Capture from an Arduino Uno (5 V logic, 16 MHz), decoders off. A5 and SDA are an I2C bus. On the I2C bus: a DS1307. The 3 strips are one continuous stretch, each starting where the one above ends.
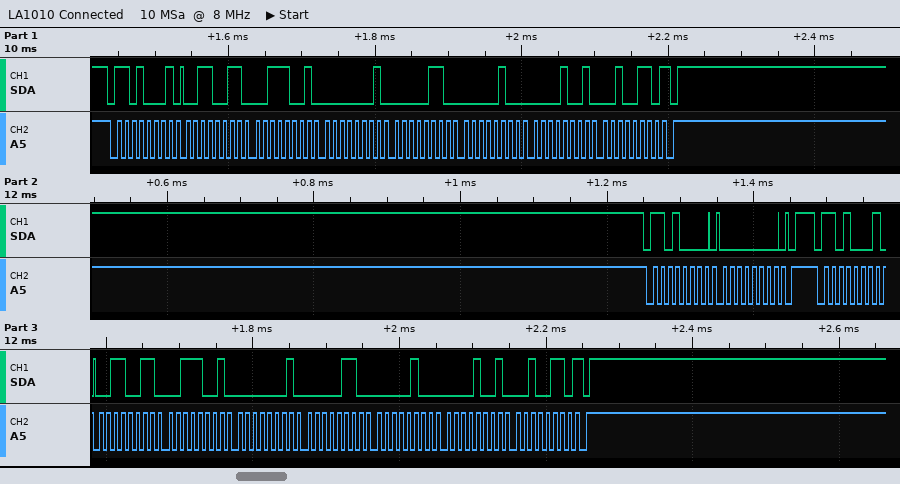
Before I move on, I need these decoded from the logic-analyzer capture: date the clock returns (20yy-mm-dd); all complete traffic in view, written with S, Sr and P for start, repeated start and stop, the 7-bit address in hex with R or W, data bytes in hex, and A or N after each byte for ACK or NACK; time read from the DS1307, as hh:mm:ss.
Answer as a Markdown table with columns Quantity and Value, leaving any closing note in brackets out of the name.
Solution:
| Quantity | Value |
|---|---|
| date the clock returns | 2026-09-04 |
| all complete traffic in view, written with S, Sr and P for start, repeated start and stop, the 7-bit address in hex with R or W, data bytes in hex, and A or N after each byte for ACK or NACK | S 68R A 33 A 39 A 01 A 06 A 04 A 09 A 26 N P S 68W A 00 A P S 68R A 33 A 39 A 01 A 06 A 04 A 09 A 26 N P |
| time read from the DS1307, as hh:mm:ss | 01:39:33 |
